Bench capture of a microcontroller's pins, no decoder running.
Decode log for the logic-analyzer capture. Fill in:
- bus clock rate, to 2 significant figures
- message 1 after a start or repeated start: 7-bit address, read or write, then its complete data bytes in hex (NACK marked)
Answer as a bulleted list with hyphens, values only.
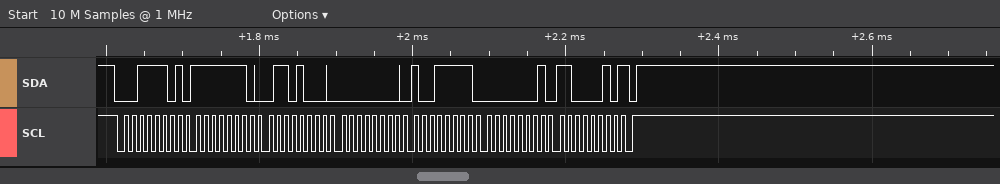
- 100 kHz
- 0x1E read: FE 68 00 9F 01 C2 NACK
